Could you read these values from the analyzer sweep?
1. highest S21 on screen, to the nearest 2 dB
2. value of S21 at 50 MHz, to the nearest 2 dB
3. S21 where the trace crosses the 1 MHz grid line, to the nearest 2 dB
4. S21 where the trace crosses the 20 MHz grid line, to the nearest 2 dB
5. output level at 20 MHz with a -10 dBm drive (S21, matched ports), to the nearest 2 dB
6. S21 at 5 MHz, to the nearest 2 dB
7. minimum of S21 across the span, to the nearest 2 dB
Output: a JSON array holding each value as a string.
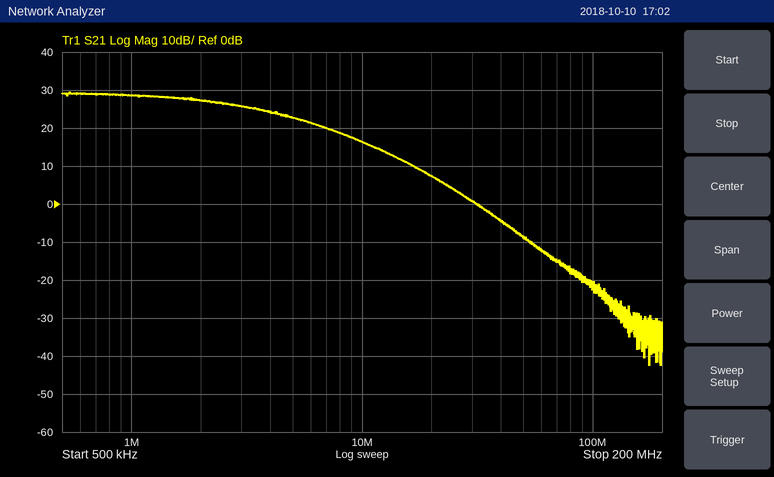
["30 dB", "-8 dB", "28 dB", "8 dB", "-2 dBm", "22 dB", "-42 dB"]
